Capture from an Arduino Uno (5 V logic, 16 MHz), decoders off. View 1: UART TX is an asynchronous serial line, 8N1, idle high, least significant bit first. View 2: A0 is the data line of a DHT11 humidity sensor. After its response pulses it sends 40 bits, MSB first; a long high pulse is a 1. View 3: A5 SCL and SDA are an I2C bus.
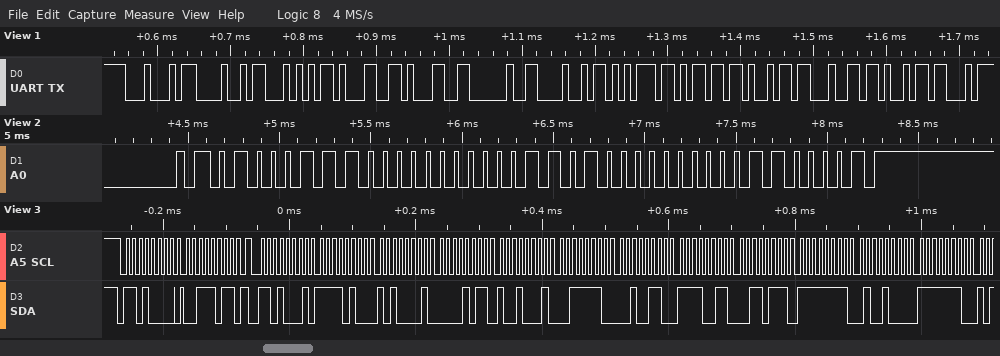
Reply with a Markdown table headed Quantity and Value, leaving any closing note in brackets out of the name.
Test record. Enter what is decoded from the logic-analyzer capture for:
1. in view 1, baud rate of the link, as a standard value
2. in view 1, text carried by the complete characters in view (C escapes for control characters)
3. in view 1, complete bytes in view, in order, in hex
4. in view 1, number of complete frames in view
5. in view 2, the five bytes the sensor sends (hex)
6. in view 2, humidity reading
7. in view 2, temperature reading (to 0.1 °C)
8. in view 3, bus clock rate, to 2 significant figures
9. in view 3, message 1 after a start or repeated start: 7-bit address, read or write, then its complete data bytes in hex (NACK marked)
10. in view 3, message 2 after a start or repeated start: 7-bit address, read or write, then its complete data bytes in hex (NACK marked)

| Quantity | Value |
|---|---|
| in view 1, baud rate of the link, as a standard value | 115200 baud |
| in view 1, text carried by the complete characters in view | "DHT11 Humidi" |
| in view 1, complete bytes in view, in order, in hex | 44 48 54 31 31 20 48 75 6D 69 64 69 |
| in view 1, number of complete frames in view | 12 |
| in view 2, the five bytes the sensor sends | 47 00 1A 00 61 |
| in view 2, humidity reading | 71 % |
| in view 2, temperature reading | 26.0 °C |
| in view 3, bus clock rate, to 2 significant figures | 100 kHz |
| in view 3, message 1 after a start or repeated start: 7-bit address, read or write, then its complete data bytes in hex | 0x68 write: 3B |
| in view 3, message 2 after a start or repeated start: 7-bit address, read or write, then its complete data bytes in hex | 0x68 read: F4 A1 0B 91 3E 26 F3 37 FF 48 FE |
